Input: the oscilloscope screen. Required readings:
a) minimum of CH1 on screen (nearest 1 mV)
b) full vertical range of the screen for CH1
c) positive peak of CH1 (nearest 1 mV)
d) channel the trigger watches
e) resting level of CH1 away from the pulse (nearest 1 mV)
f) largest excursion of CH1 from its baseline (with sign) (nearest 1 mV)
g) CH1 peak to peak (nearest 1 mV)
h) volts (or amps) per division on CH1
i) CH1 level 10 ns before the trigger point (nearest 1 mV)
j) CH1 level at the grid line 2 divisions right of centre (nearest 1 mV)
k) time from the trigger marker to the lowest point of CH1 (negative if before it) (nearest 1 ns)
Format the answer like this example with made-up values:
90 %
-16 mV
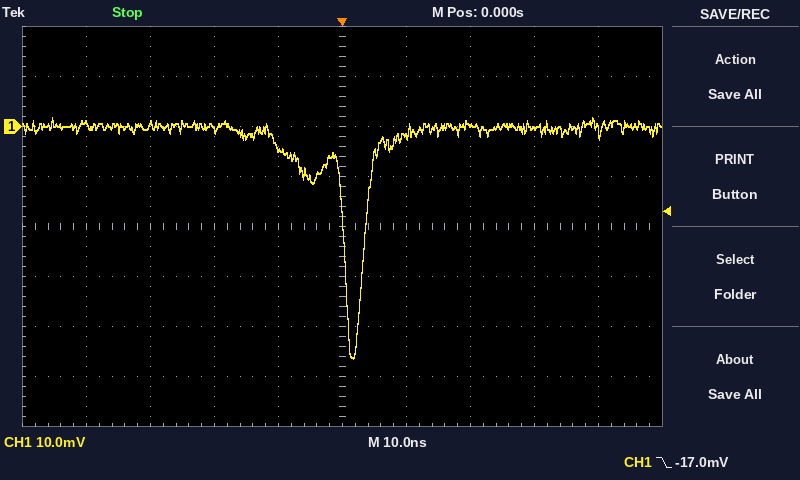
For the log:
-46 mV
80 mV
2 mV
CH1
0 mV
-46 mV
48 mV
10 mV
-4 mV
0 mV
+2 ns
